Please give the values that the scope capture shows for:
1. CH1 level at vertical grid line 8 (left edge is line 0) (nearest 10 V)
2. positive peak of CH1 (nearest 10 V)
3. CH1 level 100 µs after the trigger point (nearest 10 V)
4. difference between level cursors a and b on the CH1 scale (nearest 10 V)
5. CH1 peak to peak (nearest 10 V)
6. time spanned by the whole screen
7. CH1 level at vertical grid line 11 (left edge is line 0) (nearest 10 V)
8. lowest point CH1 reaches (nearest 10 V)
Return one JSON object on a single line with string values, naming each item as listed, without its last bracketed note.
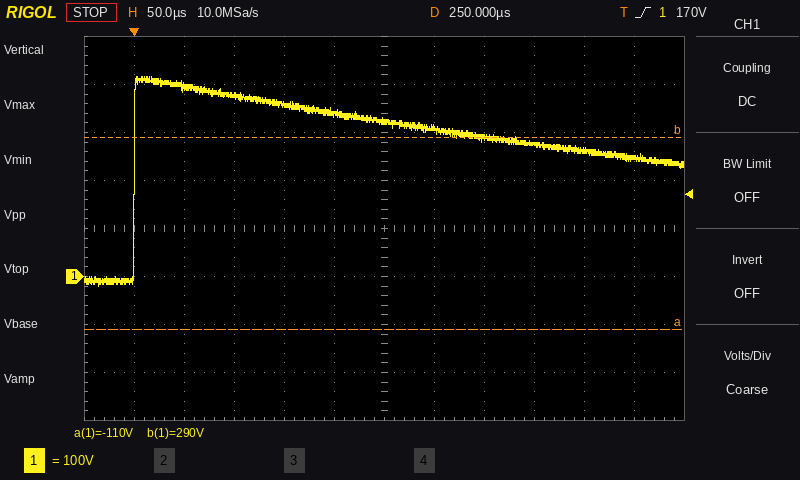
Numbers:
{"CH1 level at vertical grid line 8 (left edge is line 0)": "290 V", "positive peak of CH1": "420 V", "CH1 level 100 µs after the trigger point": "380 V", "difference between level cursors a and b on the CH1 scale": "400 V", "CH1 peak to peak": "440 V", "time spanned by the whole screen": "600 µs", "CH1 level at vertical grid line 11 (left edge is line 0)": "250 V", "lowest point CH1 reaches": "-20 V"}
